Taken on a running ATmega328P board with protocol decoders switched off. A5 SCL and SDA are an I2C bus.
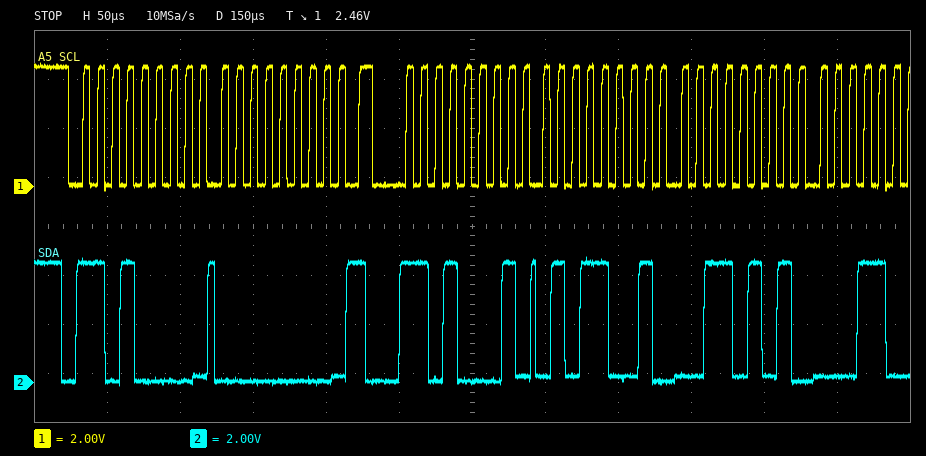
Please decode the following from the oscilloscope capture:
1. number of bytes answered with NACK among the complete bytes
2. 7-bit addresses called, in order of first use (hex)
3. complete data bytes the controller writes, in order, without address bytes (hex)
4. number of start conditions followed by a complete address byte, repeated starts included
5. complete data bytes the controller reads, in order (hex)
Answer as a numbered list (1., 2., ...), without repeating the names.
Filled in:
1. 0
2. 0x68
3. 00
4. 2
5. 59 35
